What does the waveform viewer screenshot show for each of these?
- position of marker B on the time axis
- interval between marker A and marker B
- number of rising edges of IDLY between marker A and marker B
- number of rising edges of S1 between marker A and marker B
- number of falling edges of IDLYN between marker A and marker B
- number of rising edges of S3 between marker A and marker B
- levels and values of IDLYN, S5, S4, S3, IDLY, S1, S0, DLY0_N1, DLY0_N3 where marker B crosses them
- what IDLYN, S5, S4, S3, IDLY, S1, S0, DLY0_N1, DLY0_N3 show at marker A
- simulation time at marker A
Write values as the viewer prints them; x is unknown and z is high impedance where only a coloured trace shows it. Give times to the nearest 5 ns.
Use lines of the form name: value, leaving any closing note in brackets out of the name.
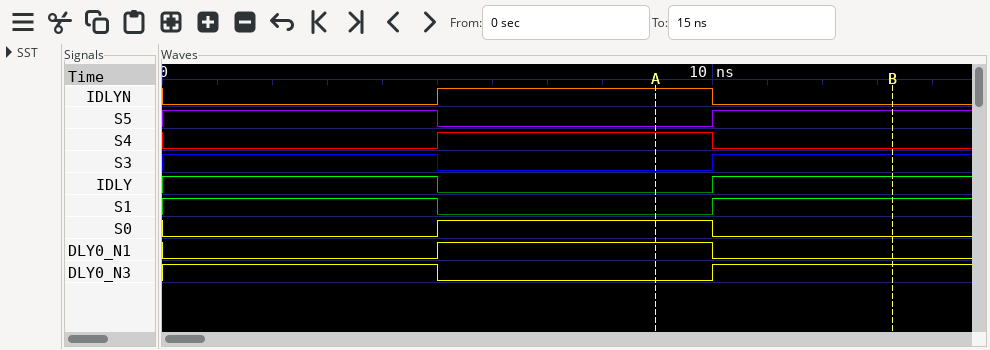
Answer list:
position of marker B on the time axis: 15 ns
interval between marker A and marker B: 5 ns
number of rising edges of IDLY between marker A and marker B: 1
number of rising edges of S1 between marker A and marker B: 1
number of falling edges of IDLYN between marker A and marker B: 1
number of rising edges of S3 between marker A and marker B: 1
levels and values of IDLYN, S5, S4, S3, IDLY, S1, S0, DLY0_N1, DLY0_N3 where marker B crosses them: IDLYN=0, S5=1, S4=0, S3=1, IDLY=1, S1=1, S0=0, DLY0_N1=0, DLY0_N3=1
what IDLYN, S5, S4, S3, IDLY, S1, S0, DLY0_N1, DLY0_N3 show at marker A: IDLYN=1, S5=0, S4=1, S3=0, IDLY=0, S1=0, S0=1, DLY0_N1=1, DLY0_N3=0
simulation time at marker A: 10 ns
